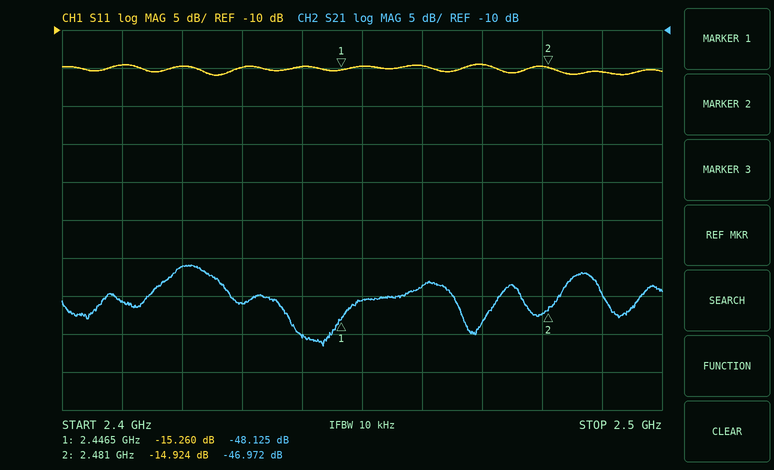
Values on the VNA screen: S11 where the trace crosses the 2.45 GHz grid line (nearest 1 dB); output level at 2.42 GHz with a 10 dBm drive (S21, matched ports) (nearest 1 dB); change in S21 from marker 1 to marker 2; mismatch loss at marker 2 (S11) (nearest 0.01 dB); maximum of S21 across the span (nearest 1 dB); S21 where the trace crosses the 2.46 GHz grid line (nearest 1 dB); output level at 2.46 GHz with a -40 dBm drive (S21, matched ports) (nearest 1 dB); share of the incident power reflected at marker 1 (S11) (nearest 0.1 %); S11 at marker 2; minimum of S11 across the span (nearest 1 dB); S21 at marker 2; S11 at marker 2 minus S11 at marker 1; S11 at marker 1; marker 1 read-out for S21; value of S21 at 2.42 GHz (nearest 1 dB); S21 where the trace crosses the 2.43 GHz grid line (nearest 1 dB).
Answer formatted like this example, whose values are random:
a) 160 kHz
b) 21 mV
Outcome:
a) -15 dB
b) -31 dBm
c) 1.153 dB
d) 0.14 dB
e) -41 dB
f) -44 dB
g) -84 dBm
h) 3.0 %
i) -14.924 dB
j) -16 dB
k) -46.972 dB
l) 0.336 dB
m) -15.260 dB
n) -48.125 dB
o) -41 dB
p) -46 dB
